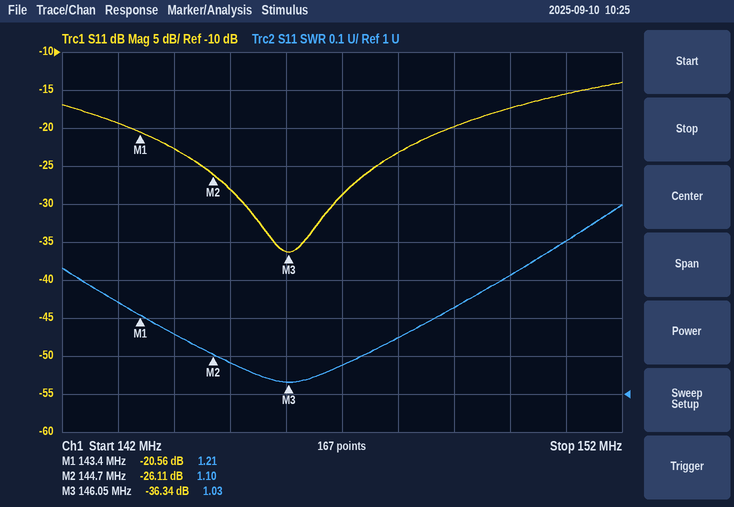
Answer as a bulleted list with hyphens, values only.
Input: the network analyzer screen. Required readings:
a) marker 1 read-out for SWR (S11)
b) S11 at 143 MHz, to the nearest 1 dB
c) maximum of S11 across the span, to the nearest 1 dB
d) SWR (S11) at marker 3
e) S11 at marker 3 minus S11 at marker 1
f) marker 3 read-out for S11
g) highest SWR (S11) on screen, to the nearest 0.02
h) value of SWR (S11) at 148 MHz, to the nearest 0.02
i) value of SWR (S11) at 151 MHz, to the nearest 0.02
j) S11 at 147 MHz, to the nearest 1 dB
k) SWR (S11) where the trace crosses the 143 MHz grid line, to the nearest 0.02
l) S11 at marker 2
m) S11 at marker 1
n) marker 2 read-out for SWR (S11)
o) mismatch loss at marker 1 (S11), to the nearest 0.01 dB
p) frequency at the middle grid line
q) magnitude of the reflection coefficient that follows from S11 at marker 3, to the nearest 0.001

- 1.21
- -19 dB
- -14 dB
- 1.03
- -15.78 dB
- -36.34 dB
- 1.50
- 1.14
- 1.40
- -29 dB
- 1.24
- -26.11 dB
- -20.56 dB
- 1.10
- 0.04 dB
- 147 MHz
- 0.015
